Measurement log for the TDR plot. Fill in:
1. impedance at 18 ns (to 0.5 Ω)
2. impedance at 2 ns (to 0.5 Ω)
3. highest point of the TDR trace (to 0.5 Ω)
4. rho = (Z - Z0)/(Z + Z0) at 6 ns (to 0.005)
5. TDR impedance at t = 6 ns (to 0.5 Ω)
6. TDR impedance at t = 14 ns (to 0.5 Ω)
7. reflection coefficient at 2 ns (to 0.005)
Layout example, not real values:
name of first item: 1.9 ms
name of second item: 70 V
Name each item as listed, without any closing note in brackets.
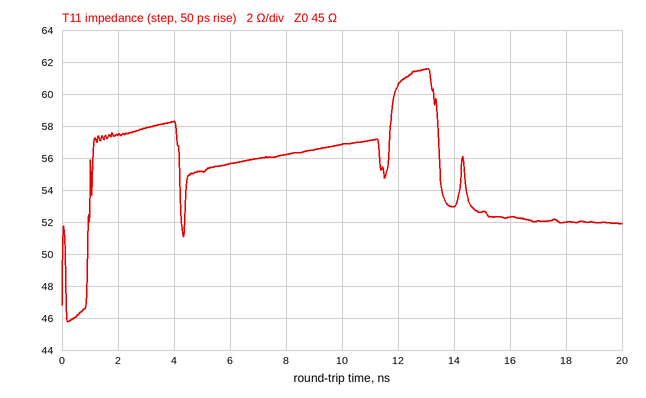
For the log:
impedance at 18 ns: 52.0 Ω
impedance at 2 ns: 57.5 Ω
highest point of the TDR trace: 61.5 Ω
rho = (Z - Z0)/(Z + Z0) at 6 ns: +0.105
TDR impedance at t = 6 ns: 55.5 Ω
TDR impedance at t = 14 ns: 53.0 Ω
reflection coefficient at 2 ns: +0.120
